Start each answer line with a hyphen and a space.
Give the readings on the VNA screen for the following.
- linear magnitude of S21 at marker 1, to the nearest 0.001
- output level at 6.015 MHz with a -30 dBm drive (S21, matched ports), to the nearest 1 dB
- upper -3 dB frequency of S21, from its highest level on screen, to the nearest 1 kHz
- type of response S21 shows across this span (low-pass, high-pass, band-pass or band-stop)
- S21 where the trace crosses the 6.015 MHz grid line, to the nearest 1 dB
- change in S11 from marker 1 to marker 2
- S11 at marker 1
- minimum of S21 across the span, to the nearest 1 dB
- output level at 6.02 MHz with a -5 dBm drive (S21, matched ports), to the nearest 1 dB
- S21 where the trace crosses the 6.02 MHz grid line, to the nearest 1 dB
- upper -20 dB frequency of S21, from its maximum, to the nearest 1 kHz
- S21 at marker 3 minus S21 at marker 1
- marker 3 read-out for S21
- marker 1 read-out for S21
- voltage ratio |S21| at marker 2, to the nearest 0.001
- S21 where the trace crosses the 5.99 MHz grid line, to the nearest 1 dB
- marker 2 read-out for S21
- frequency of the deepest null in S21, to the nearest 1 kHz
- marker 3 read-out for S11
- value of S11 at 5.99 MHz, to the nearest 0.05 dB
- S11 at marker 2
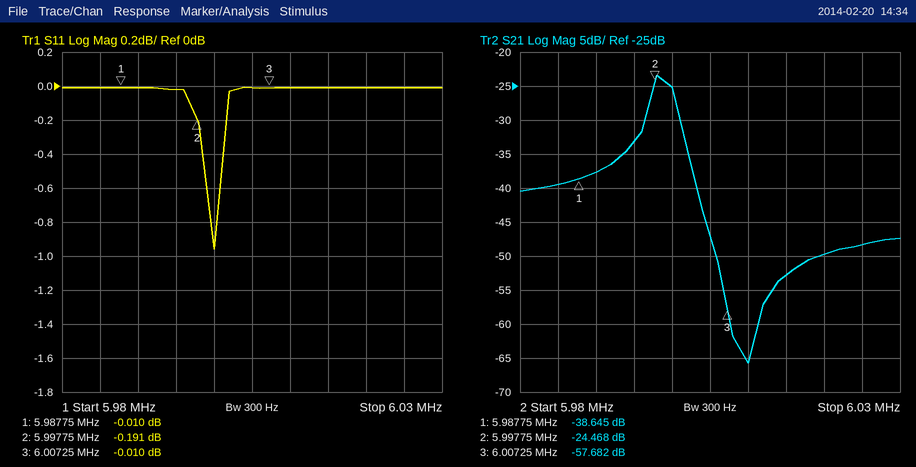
- 0.012
- -83 dBm
- 6.000 MHz
- band-pass
- -53 dB
- -0.181 dB
- -0.010 dB
- -66 dB
- -55 dBm
- -50 dB
- 6.004 MHz
- -19.037 dB
- -57.682 dB
- -38.645 dB
- 0.060
- -38 dB
- -24.468 dB
- 6.010 MHz
- -0.010 dB
- 0.00 dB
- -0.191 dB
